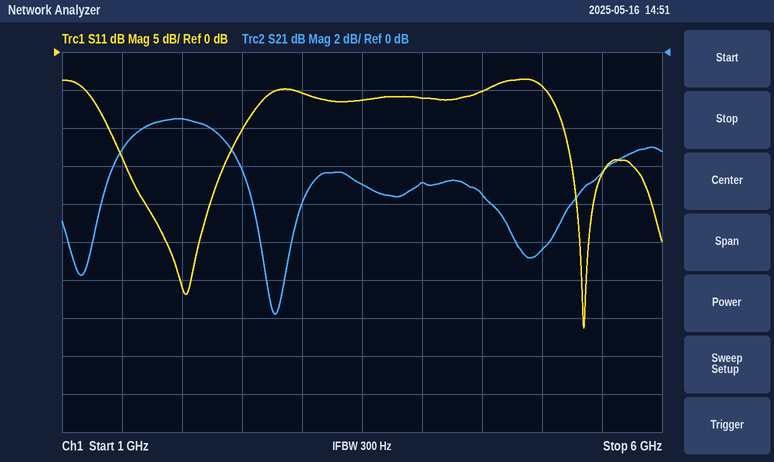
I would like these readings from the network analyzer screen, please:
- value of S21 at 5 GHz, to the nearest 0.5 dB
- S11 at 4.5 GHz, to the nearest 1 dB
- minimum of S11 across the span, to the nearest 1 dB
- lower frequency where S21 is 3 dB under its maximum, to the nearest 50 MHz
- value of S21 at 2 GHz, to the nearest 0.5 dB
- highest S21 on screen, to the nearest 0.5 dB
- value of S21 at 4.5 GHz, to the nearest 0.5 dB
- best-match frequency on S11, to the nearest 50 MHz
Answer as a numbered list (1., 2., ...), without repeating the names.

1. -10.5 dB
2. -5 dB
3. -36 dB
4. 1.40 GHz
5. -3.5 dB
6. -3.5 dB
7. -7.5 dB
8. 5.35 GHz
